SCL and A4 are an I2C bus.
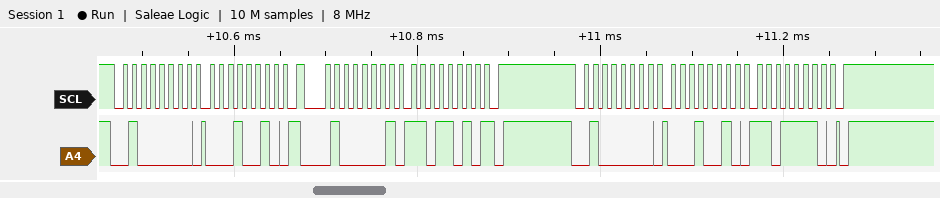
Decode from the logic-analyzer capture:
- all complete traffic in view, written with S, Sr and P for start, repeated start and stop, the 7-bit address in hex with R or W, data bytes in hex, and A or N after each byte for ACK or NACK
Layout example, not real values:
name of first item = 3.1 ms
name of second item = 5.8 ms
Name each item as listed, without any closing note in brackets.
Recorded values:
all complete traffic in view, written with S, Sr and P for start, repeated start and stop, the 7-bit address in hex with R or W, data bytes in hex, and A or N after each byte for ACK or NACK = S 20W A 12 A Sr 20R A DA N P S 20W A 12 A DE A P
